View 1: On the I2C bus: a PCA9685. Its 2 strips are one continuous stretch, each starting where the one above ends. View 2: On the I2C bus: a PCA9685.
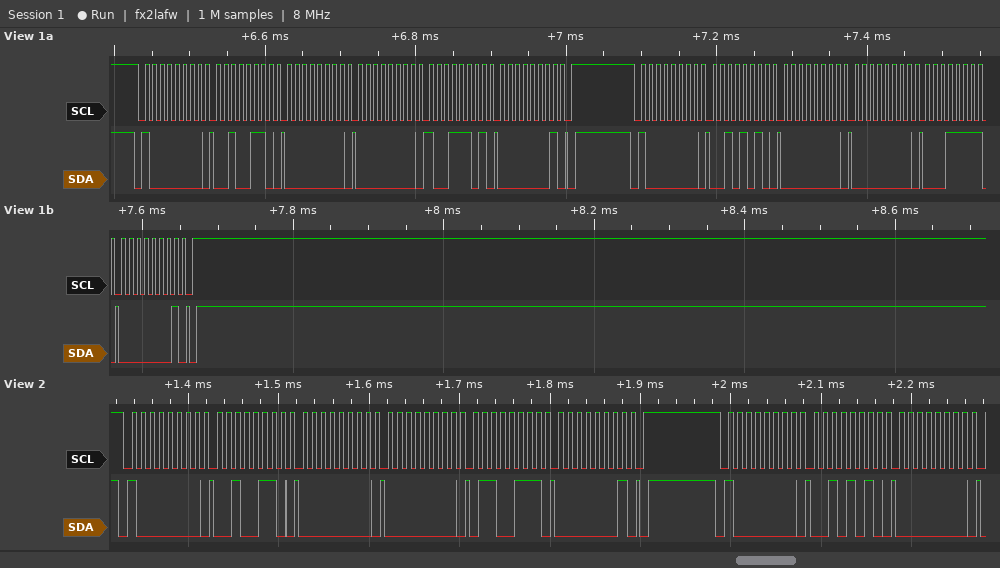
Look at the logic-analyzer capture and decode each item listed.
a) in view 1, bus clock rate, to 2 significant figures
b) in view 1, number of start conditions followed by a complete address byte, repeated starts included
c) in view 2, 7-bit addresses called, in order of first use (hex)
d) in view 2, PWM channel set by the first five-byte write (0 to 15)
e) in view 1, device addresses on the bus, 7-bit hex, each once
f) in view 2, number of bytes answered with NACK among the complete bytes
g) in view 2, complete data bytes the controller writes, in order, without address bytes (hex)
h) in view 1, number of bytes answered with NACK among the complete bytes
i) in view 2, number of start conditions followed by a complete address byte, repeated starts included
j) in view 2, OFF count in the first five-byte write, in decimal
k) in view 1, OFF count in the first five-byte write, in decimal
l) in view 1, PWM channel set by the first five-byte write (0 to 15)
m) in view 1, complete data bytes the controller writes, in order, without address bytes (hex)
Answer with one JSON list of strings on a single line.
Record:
["100 kHz", "2", "0x40", "8", "0x40", "0", "26 00 00 67 01 2A 00", "0", "2", "359", "413", "8", "26 00 00 9D 01 2A 00 00 1F 01"]
